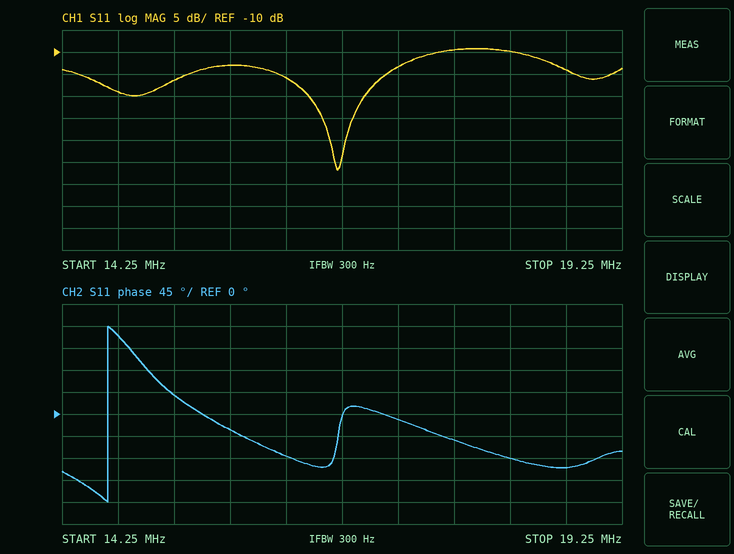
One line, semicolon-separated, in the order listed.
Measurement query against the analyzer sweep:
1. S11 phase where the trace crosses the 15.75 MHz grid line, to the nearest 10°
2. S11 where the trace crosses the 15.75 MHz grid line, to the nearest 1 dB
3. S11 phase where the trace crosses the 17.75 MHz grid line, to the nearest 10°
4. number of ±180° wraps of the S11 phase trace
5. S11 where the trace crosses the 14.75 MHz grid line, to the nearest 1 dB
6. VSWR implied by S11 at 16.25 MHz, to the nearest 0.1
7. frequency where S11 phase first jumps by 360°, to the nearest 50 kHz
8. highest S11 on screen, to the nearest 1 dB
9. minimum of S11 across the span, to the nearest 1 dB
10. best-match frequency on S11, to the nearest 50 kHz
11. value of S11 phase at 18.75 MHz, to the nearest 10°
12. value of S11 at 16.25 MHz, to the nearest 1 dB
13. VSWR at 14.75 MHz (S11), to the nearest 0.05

-30°; -13 dB; -50°; 1; -19 dB; 1.4; 14.65 MHz; -9 dB; -37 dB; 16.70 MHz; -110°; -16 dB; 1.25
